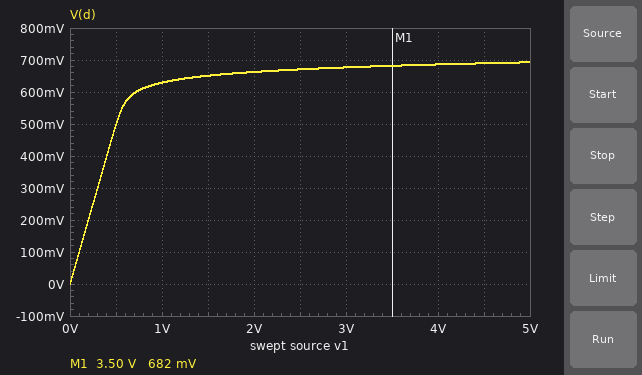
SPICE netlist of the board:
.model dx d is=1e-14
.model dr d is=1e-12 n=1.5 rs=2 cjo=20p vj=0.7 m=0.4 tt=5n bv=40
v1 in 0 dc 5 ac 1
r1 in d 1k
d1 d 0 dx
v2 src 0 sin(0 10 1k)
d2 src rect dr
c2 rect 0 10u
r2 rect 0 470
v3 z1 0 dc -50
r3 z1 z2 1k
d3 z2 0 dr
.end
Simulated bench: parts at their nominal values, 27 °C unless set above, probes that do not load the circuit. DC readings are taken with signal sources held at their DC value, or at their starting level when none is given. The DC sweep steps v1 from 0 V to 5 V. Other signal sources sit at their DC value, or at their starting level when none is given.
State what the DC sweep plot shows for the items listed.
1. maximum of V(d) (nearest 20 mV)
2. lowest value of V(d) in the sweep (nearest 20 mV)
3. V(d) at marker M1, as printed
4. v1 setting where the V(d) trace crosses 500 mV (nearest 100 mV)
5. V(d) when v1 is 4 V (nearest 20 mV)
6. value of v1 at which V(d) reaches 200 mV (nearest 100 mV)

700 mV
0 V
682 mV
500 mV
680 mV
200 mV
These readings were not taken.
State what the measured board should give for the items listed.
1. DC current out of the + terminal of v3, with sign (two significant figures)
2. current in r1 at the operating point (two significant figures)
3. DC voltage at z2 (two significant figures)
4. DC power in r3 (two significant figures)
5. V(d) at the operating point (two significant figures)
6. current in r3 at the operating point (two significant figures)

-9.9 mA
4.3 mA
-40 V
98 mW
690 mV
9.9 mA
